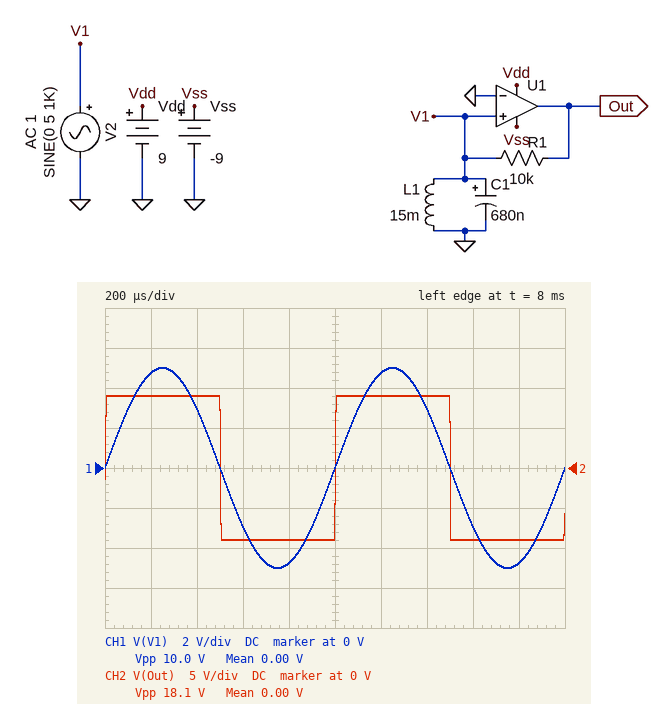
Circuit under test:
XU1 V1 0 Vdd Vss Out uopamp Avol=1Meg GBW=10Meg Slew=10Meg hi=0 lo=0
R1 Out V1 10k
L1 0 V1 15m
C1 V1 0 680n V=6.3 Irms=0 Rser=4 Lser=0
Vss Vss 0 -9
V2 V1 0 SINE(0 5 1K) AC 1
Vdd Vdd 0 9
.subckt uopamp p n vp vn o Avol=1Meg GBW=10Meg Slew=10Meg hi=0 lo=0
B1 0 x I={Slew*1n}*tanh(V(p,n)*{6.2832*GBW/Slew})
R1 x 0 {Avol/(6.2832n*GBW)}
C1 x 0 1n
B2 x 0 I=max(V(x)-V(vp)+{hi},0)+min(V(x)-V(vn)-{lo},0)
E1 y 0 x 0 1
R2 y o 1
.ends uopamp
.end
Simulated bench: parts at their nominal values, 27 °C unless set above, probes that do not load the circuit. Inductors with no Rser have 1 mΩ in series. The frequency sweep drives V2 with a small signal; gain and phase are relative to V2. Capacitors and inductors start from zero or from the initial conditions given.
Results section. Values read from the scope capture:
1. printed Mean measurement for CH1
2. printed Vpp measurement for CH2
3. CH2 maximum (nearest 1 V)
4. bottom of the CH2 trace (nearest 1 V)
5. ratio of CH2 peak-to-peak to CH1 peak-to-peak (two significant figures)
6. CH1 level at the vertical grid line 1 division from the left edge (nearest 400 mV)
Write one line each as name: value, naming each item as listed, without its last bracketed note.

printed Mean measurement for CH1: 0.00 V
printed Vpp measurement for CH2: 18.1 V
CH2 maximum: 9 V
bottom of the CH2 trace: -9 V
ratio of CH2 peak-to-peak to CH1 peak-to-peak: 1.8
CH1 level at the vertical grid line 1 division from the left edge: 4.8 V
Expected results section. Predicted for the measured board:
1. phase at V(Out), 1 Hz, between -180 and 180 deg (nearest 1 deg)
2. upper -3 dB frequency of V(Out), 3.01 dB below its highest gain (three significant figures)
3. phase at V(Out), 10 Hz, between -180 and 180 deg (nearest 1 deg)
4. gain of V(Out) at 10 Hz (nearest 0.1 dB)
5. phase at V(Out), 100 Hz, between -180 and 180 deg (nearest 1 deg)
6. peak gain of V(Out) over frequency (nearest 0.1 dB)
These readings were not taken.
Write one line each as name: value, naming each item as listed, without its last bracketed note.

phase at V(Out), 1 Hz, between -180 and 180 deg: -6 deg
upper -3 dB frequency of V(Out), 3.01 dB below its highest gain: 10.0 Hz
phase at V(Out), 10 Hz, between -180 and 180 deg: -45 deg
gain of V(Out) at 10 Hz: 117.0 dB
phase at V(Out), 100 Hz, between -180 and 180 deg: -84 deg
peak gain of V(Out) over frequency: 120.0 dB
